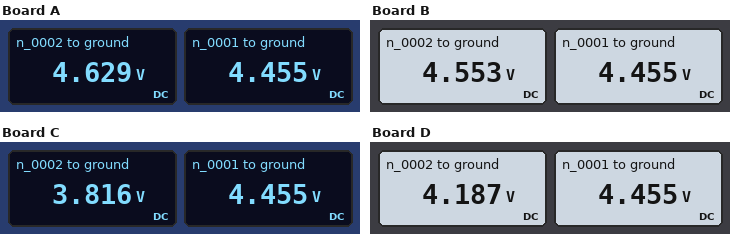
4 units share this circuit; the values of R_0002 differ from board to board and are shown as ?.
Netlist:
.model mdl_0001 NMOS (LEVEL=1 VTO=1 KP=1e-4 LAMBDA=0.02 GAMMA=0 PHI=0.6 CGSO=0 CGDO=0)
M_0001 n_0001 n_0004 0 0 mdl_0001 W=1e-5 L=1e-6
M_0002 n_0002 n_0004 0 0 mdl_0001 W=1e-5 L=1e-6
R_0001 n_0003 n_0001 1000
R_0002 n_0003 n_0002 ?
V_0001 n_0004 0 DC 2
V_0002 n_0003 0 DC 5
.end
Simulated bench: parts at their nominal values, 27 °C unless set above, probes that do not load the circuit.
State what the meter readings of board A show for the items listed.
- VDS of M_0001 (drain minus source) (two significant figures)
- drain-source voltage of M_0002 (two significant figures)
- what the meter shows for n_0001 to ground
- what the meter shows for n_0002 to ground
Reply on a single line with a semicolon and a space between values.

4.5 V; 4.6 V; 4.455 V; 4.629 V
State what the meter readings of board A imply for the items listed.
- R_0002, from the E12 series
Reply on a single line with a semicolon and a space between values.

680 Ω
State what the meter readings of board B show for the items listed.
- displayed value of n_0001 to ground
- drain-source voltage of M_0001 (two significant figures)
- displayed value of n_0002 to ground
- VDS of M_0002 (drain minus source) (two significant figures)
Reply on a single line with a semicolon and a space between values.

4.455 V; 4.5 V; 4.553 V; 4.6 V
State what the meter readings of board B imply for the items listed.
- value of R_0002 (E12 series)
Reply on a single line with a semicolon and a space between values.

820 Ω
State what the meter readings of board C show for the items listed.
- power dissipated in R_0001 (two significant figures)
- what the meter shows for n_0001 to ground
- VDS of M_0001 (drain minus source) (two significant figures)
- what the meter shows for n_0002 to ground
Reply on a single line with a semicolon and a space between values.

300 µW; 4.455 V; 4.5 V; 3.816 V
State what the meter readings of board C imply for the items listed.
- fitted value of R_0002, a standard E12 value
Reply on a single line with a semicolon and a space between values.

2.2 kΩ
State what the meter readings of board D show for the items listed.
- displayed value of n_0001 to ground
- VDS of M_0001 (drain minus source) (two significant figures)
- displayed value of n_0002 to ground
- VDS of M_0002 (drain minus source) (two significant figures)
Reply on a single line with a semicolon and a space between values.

4.455 V; 4.5 V; 4.187 V; 4.2 V
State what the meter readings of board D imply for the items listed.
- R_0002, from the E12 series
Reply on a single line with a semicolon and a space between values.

1.5 kΩ
